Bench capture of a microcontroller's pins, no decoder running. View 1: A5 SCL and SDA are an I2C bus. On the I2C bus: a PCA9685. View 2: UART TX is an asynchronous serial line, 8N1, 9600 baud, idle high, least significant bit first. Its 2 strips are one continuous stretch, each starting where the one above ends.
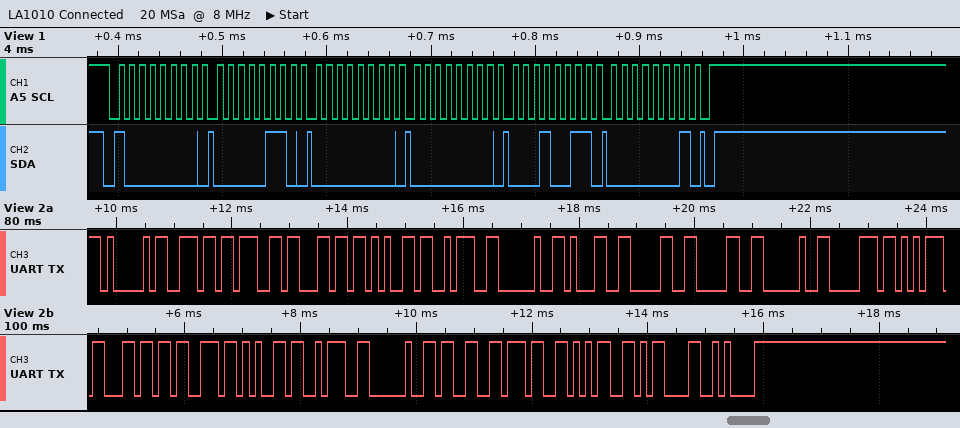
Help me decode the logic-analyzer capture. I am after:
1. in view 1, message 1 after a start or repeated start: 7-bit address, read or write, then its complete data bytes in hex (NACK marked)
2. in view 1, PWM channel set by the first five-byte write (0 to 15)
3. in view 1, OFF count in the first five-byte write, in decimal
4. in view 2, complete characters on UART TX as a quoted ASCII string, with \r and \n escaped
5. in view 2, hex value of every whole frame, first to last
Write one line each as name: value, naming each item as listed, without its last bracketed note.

in view 1, message 1 after a start or repeated start: 7-bit address, read or write, then its complete data bytes in hex: 0x40 write: 06 00 00 13 01
in view 1, PWM channel set by the first five-byte write: 0
in view 1, OFF count in the first five-byte write, in decimal: 275
in view 2, complete characters on UART TX as a quoted ASCII string, with \r and \n escaped: "Angle: 100 pulse: 375\r\n"
in view 2, hex value of every whole frame, first to last: 0x41 0x6E 0x67 0x6C 0x65 0x3A 0x20 0x31 0x30 0x30 0x20 0x70 0x75 0x6C 0x73 0x65 0x3A 0x20 0x33 0x37 0x35 0x0D 0x0A
